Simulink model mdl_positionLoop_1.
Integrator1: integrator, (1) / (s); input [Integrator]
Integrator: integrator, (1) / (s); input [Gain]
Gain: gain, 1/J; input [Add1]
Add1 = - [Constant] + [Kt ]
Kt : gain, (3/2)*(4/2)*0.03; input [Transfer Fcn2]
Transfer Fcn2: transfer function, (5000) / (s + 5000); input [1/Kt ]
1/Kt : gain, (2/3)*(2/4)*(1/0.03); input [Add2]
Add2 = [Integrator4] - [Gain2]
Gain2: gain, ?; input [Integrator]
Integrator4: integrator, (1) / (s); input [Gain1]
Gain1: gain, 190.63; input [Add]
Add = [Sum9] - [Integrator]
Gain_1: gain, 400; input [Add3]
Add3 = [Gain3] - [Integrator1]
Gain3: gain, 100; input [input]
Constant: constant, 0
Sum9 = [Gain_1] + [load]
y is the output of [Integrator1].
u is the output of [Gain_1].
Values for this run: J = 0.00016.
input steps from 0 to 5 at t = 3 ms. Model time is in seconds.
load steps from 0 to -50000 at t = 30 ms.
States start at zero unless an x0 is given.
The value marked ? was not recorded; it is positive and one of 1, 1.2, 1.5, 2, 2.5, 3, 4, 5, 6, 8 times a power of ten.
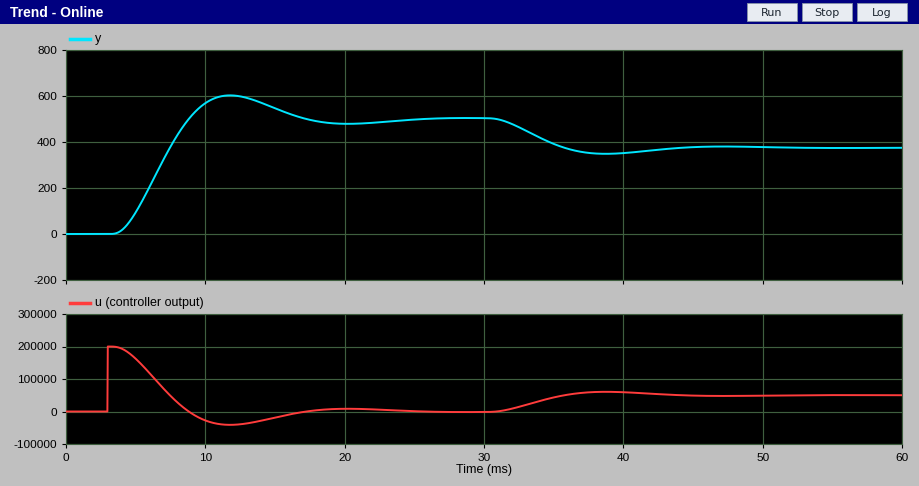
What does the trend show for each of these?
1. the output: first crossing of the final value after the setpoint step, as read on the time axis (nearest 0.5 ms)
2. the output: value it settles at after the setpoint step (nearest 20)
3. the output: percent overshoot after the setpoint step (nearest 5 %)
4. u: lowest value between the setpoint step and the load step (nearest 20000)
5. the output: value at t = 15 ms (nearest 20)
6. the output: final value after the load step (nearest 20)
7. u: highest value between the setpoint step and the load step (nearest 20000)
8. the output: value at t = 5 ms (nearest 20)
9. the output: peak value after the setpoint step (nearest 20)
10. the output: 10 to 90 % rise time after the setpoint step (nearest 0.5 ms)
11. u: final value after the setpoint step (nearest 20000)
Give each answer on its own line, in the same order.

9.0 ms
500
20 %
-40000
540
380
200000
100
600
3.5 ms
0
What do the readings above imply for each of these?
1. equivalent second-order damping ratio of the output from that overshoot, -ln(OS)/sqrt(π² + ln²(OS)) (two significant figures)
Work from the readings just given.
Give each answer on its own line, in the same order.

0.46
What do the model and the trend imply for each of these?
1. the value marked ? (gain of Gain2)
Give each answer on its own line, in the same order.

0.5
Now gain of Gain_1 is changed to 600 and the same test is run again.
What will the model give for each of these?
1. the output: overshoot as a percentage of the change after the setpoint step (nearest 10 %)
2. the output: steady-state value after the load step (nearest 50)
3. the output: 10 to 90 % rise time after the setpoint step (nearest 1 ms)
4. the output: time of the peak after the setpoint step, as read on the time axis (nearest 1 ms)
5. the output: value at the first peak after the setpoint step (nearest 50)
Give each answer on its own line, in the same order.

30 %
400
3 ms
10 ms
650
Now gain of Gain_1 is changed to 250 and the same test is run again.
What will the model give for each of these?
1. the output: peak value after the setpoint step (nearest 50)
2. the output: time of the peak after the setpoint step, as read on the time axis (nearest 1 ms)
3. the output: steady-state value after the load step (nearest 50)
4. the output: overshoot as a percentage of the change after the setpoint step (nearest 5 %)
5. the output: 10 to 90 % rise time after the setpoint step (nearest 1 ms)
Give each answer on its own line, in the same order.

550
15 ms
300
10 %
6 ms
